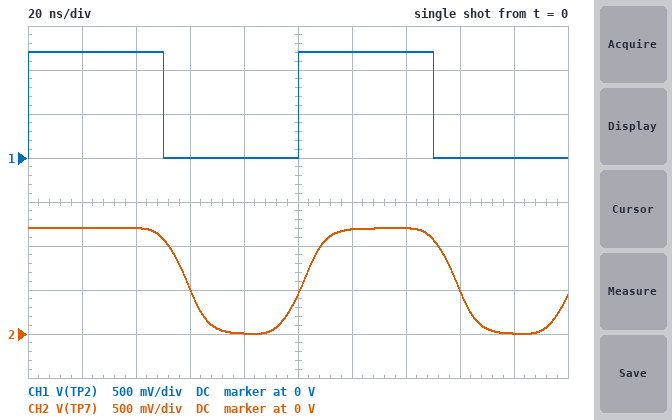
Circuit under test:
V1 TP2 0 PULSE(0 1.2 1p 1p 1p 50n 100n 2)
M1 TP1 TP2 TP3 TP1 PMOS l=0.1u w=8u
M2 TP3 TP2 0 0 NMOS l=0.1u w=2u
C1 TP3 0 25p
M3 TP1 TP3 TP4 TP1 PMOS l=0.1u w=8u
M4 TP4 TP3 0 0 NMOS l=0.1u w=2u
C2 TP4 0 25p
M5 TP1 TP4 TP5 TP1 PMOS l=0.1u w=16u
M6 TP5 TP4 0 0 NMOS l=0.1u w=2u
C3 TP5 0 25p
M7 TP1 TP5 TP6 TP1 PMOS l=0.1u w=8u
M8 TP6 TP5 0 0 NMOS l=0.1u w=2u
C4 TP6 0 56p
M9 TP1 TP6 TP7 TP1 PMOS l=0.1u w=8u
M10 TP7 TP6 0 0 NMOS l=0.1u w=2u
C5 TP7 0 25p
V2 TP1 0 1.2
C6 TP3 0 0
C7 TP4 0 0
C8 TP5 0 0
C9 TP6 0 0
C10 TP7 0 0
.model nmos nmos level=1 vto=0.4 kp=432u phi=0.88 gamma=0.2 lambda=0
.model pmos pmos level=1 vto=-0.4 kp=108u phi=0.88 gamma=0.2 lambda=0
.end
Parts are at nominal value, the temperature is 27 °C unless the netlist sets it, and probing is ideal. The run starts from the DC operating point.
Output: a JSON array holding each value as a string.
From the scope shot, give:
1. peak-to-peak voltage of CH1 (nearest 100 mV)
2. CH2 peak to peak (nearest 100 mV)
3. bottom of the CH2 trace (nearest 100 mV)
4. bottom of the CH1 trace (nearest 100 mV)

["1.2 V", "1.2 V", "0 V", "0 V"]
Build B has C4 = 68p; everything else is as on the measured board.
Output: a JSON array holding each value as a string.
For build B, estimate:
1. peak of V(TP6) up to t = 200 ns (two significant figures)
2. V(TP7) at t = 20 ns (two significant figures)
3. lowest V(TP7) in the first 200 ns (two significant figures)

["1.1 V", "1.2 V", "7.0 mV"]
